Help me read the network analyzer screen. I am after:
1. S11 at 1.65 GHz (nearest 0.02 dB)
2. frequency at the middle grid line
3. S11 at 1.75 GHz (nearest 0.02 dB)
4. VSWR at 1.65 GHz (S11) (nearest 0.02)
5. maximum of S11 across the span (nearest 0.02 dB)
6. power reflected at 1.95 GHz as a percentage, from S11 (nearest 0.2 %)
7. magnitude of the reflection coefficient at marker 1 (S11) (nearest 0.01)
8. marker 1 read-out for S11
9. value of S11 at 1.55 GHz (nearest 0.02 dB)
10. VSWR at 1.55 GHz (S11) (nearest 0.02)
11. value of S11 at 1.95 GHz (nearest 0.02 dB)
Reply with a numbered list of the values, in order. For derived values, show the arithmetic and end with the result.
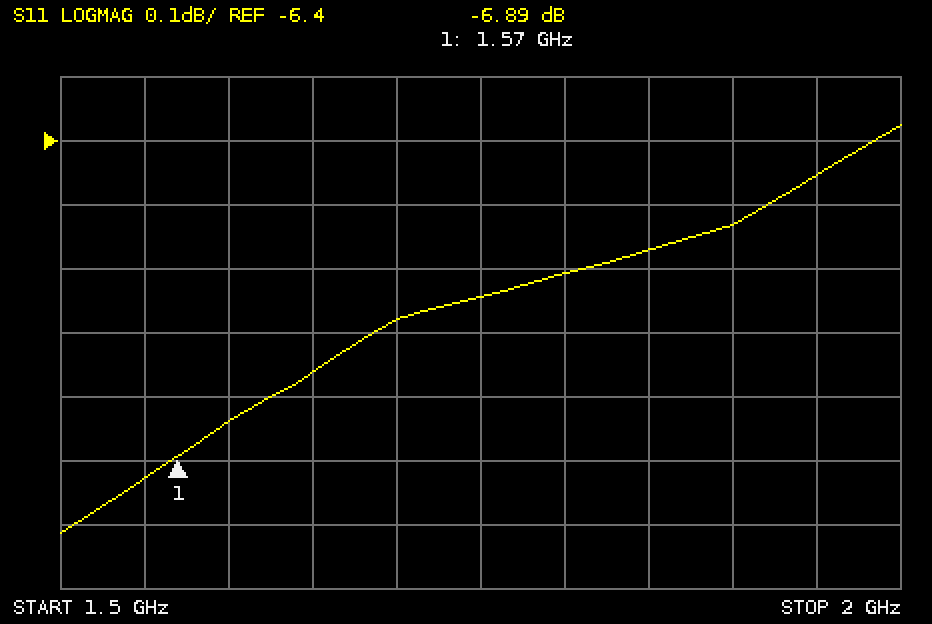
1. -6.76 dB
2. 1.75 GHz
3. -6.64 dB
4. |Γ| = 10^(-6.76/20) = 0.4592; VSWR = (1 + 0.4592)/(1 − 0.4592) ≈ 2.70
5. -6.38 dB
6. 10^(-6.46/10) ≈ 22.6 %
7. 10^(-6.89/20) ≈ 0.45
8. -6.89 dB
9. -6.92 dB
10. |Γ| = 10^(-6.92/20) = 0.4508; VSWR = (1 + 0.4508)/(1 − 0.4508) ≈ 2.64
11. -6.46 dB
